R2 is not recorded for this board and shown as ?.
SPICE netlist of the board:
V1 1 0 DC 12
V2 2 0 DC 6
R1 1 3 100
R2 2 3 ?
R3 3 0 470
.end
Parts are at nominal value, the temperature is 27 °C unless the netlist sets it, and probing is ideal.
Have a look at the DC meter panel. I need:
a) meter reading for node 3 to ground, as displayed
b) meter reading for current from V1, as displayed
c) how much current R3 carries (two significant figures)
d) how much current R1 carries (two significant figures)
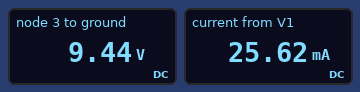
9.44 V
25.62 mA
20 mA
26 mA
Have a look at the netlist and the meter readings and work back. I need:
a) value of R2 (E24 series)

620 Ω
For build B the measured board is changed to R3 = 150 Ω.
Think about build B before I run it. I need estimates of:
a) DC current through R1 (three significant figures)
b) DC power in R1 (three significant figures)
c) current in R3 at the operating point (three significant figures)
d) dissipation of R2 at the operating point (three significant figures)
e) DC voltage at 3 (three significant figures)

49.1 mA
241 mW
47.3 mA
1.93 mW
7.09 V
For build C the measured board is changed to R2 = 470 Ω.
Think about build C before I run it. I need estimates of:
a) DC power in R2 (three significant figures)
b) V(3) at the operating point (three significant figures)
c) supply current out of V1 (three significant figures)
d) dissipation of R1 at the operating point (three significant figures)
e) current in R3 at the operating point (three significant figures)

23.4 mW
9.31 V
26.9 mA
72.2 mW
19.8 mA
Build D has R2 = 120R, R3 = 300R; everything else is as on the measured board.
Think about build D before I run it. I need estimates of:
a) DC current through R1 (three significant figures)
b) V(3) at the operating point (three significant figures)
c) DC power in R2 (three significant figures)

41.5 mA
7.85 V
28.4 mW
